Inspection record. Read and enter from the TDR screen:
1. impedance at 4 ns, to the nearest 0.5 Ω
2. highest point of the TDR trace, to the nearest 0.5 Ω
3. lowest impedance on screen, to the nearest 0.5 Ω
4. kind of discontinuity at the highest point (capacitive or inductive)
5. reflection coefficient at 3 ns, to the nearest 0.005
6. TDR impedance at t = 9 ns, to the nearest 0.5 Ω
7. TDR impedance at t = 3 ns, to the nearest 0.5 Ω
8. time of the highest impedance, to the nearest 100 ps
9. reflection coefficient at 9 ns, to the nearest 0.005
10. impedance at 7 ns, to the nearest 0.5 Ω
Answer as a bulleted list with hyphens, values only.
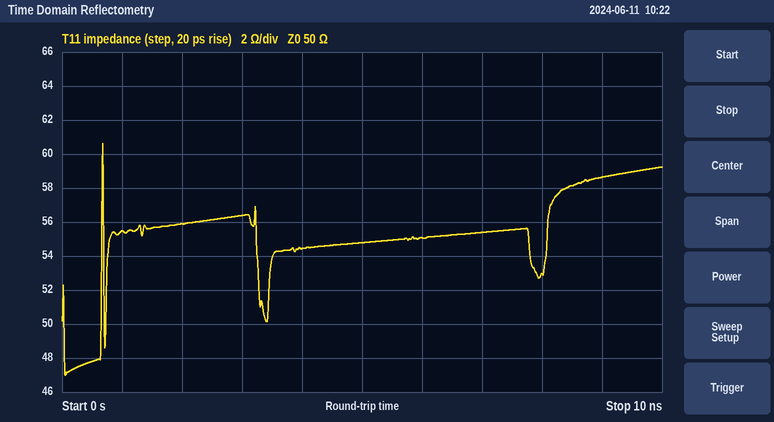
- 54.5 Ω
- 60.5 Ω
- 47.0 Ω
- inductive
- +0.060
- 58.5 Ω
- 56.5 Ω
- 700 ps
- +0.080
- 55.5 Ω
